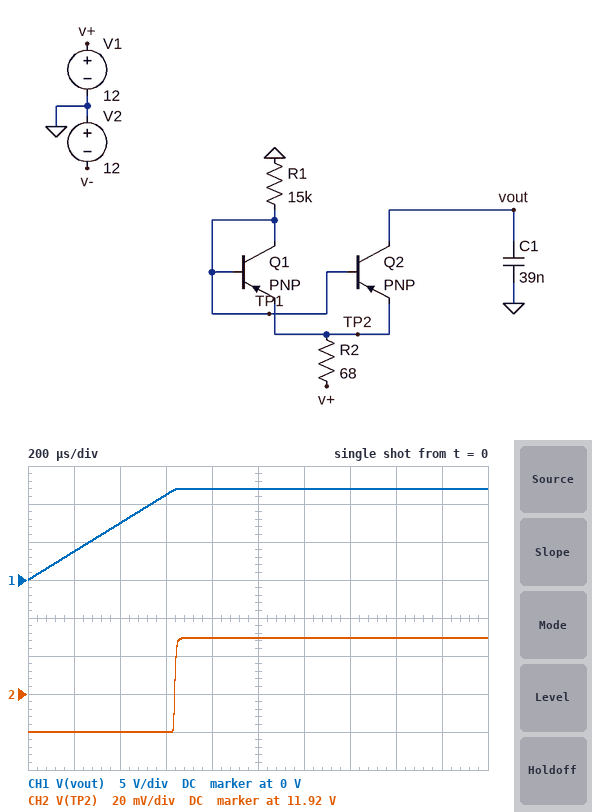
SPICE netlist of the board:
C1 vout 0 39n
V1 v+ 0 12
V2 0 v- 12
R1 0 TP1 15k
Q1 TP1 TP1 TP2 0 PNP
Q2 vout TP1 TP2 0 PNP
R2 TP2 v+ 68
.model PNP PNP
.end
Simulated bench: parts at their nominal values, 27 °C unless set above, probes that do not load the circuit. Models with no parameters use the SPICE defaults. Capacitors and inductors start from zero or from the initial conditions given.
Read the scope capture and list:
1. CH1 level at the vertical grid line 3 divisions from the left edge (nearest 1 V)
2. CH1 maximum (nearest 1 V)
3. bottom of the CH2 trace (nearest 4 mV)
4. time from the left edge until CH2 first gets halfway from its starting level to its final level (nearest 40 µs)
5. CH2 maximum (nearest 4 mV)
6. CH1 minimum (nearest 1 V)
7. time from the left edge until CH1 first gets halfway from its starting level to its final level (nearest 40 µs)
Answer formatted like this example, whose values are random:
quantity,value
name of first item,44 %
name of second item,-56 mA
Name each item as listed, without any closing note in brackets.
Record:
quantity,value
CH1 level at the vertical grid line 3 divisions from the left edge,11 V
CH1 maximum,12 V
bottom of the CH2 trace,11.900 V
time from the left edge until CH2 first gets halfway from its starting level to its final level,640 µs
CH2 maximum,11.948 V
CH1 minimum,0 V
time from the left edge until CH1 first gets halfway from its starting level to its final level,320 µs
